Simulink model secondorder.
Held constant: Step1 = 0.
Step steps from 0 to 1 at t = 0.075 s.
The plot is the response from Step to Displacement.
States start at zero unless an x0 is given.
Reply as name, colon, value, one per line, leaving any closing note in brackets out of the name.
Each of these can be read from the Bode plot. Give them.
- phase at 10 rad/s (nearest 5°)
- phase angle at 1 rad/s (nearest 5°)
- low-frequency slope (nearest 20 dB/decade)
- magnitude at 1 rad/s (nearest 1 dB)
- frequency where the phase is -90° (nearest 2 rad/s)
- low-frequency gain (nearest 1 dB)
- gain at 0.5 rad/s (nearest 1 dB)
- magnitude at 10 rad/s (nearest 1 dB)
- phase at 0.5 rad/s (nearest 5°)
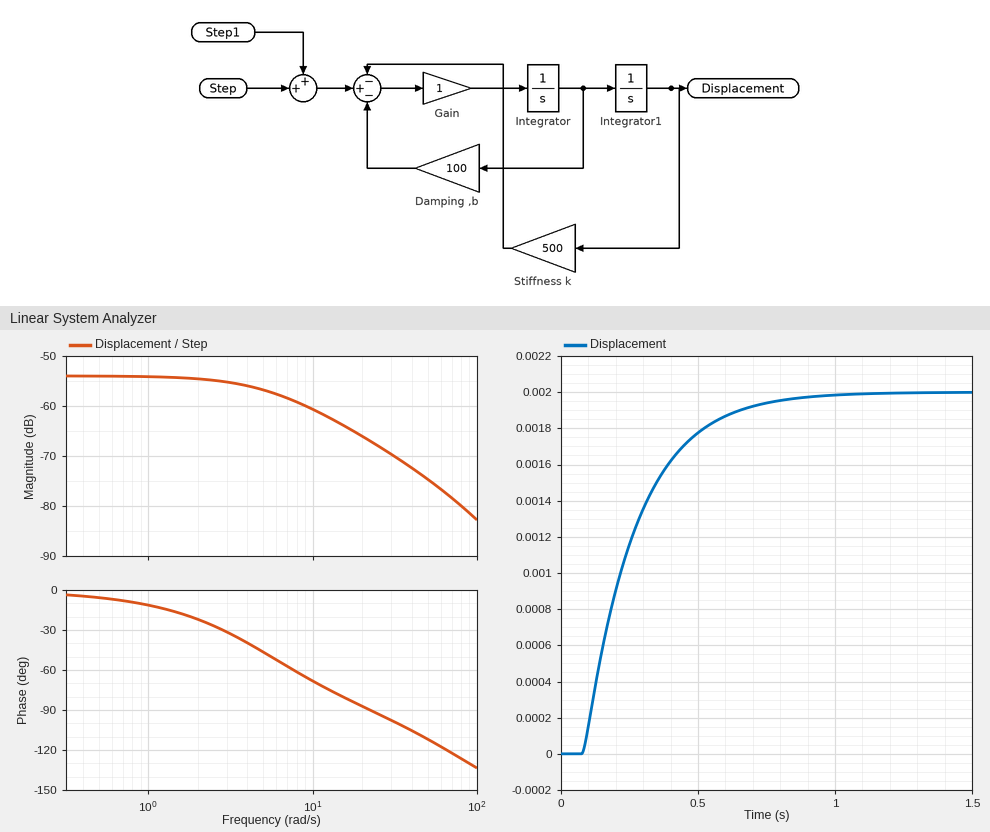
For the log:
phase at 10 rad/s: -70°
phase angle at 1 rad/s: -10°
low-frequency slope: 0 dB/decade
magnitude at 1 rad/s: -54 dB
frequency where the phase is -90°: 22 rad/s
low-frequency gain: -54 dB
gain at 0.5 rad/s: -54 dB
magnitude at 10 rad/s: -61 dB
phase at 0.5 rad/s: -5°
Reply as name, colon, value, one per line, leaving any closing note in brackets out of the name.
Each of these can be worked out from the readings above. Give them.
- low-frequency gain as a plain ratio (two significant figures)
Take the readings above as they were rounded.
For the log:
low-frequency gain as a plain ratio: 0.0020
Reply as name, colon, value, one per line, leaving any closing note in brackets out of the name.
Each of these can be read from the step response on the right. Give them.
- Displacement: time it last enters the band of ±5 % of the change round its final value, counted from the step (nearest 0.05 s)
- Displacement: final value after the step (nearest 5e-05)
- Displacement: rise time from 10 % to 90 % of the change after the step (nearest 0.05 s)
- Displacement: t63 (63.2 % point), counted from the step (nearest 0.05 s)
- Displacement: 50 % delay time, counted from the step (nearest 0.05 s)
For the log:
Displacement: time it last enters the band of ±5 % of the change round its final value, counted from the step: 0.60 s
Displacement: final value after the step: 0.00200
Displacement: rise time from 10 % to 90 % of the change after the step: 0.40 s
Displacement: t63 (63.2 % point), counted from the step: 0.20 s
Displacement: 50 % delay time, counted from the step: 0.15 s
